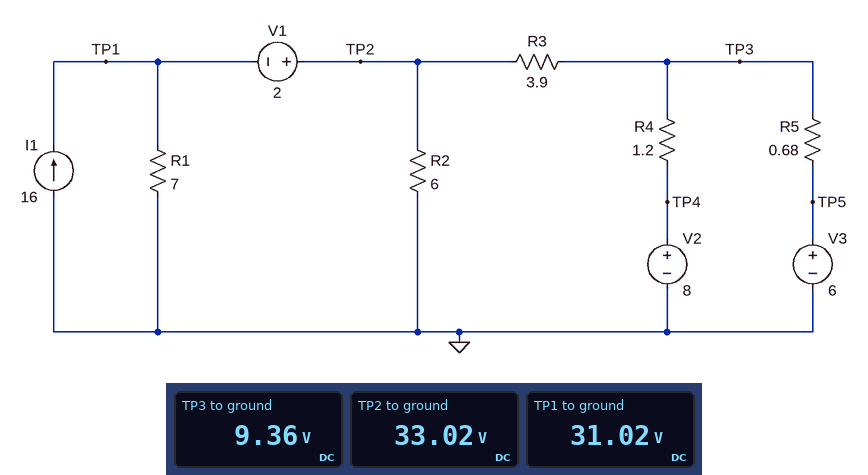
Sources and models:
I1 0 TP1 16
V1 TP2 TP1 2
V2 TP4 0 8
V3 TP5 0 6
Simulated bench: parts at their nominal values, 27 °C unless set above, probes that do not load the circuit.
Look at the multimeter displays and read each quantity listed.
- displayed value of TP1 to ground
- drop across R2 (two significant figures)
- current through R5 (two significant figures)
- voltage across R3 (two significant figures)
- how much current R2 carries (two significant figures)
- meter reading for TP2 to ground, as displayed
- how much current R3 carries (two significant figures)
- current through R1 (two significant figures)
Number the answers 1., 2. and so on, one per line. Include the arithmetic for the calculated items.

1. 31.02 V
2. 33.02 V = 33 V
3. (9.36 V - 6 V) / 680 mΩ = 4.9 A
4. 33.02 V - 9.36 V = 24 V
5. (33.02 V) / 6 Ω = 5.5 A
6. 33.02 V
7. (33.02 V - 9.36 V) / 3.9 Ω = 6.1 A
8. (31.02 V) / 7 Ω = 4.4 A
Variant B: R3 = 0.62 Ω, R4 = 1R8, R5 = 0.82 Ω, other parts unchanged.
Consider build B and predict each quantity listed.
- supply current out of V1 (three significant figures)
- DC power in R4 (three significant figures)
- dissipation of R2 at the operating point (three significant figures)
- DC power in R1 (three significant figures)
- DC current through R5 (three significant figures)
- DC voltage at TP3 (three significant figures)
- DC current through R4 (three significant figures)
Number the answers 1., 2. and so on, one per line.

1. 13.6 A
2. 11.2 W
3. 59.9 W
4. 41.1 W
5. 7.92 A
6. 12.5 V
7. 2.50 A
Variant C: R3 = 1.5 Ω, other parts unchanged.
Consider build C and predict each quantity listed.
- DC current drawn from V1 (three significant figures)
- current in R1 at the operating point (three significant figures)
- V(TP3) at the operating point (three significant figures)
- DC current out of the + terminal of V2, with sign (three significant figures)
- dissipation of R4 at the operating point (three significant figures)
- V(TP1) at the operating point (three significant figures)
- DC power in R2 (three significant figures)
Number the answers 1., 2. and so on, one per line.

1. 12.9 A
2. 3.13 A
3. 10.6 V
4. -2.15 A
5. 5.55 W
6. 21.9 V
7. 95.3 W
